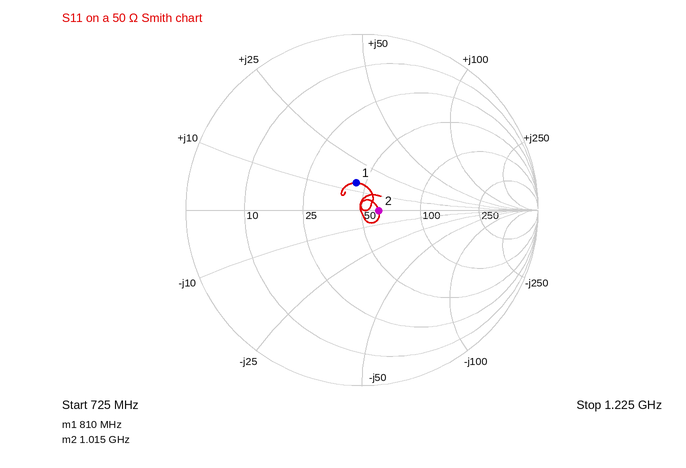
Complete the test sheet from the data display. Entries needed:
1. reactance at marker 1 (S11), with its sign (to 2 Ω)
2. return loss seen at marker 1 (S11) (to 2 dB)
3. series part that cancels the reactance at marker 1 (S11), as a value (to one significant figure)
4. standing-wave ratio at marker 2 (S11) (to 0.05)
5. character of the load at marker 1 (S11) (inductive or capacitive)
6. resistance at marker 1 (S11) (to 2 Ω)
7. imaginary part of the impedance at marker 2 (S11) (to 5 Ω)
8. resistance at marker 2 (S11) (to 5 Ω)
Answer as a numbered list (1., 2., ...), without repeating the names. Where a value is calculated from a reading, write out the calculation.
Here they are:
1. +14 Ω
2. 16 dB
3. C = 1/(2π × 810 MHz × 14 Ω) ≈ 14.0 pF, so 10 pF to one significant figure
4. 1.20
5. inductive
6. 44 Ω
7. 0 Ω
8. 60 Ω
